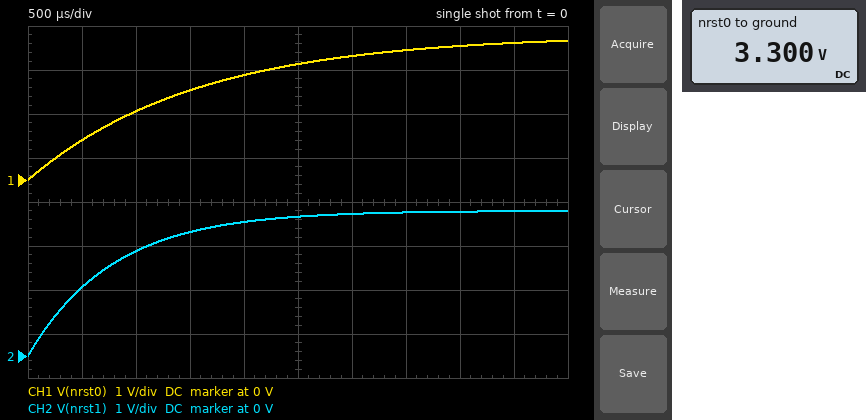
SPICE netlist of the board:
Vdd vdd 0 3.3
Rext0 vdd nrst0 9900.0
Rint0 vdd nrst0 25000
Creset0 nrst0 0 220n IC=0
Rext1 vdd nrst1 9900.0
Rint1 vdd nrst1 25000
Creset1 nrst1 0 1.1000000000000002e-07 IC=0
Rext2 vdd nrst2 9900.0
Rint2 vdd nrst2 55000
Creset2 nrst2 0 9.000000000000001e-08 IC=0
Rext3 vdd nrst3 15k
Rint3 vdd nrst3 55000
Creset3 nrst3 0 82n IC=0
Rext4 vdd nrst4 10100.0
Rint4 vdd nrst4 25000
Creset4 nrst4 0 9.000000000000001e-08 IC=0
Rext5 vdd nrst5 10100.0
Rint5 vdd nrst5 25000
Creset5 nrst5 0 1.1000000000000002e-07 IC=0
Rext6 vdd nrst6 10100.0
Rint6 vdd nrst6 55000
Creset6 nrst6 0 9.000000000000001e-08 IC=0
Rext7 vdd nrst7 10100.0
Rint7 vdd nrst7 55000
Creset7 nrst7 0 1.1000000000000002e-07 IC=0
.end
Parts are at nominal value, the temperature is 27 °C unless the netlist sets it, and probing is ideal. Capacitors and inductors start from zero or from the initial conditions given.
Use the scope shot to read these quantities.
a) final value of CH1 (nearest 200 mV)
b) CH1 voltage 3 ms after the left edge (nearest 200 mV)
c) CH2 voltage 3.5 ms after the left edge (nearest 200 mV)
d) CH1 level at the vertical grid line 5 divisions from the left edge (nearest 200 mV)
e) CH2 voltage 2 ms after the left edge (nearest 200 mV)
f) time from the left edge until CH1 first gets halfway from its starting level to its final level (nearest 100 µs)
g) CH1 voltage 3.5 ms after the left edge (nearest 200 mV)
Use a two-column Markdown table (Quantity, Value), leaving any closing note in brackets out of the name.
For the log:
| Quantity | Value |
|---|---|
| final value of CH1 | 3.2 V |
| CH1 voltage 3 ms after the left edge | 2.8 V |
| CH2 voltage 3.5 ms after the left edge | 3.2 V |
| CH1 level at the vertical grid line 5 divisions from the left edge | 2.6 V |
| CH2 voltage 2 ms after the left edge | 3.0 V |
| time from the left edge until CH1 first gets halfway from its starting level to its final level | 1.0 ms |
| CH1 voltage 3.5 ms after the left edge | 3.0 V |
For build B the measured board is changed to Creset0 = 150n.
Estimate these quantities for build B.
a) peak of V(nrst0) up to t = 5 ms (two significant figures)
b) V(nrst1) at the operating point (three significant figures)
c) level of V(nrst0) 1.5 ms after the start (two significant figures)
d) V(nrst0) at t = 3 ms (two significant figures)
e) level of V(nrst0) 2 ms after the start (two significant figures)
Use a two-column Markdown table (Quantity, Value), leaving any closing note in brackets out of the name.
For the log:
| Quantity | Value |
|---|---|
| peak of V(nrst0) up to t = 5 ms | 3.3 V |
| V(nrst1) at the operating point | 3.30 V |
| level of V(nrst0) 1.5 ms after the start | 2.5 V |
| V(nrst0) at t = 3 ms | 3.1 V |
| level of V(nrst0) 2 ms after the start | 2.8 V |
